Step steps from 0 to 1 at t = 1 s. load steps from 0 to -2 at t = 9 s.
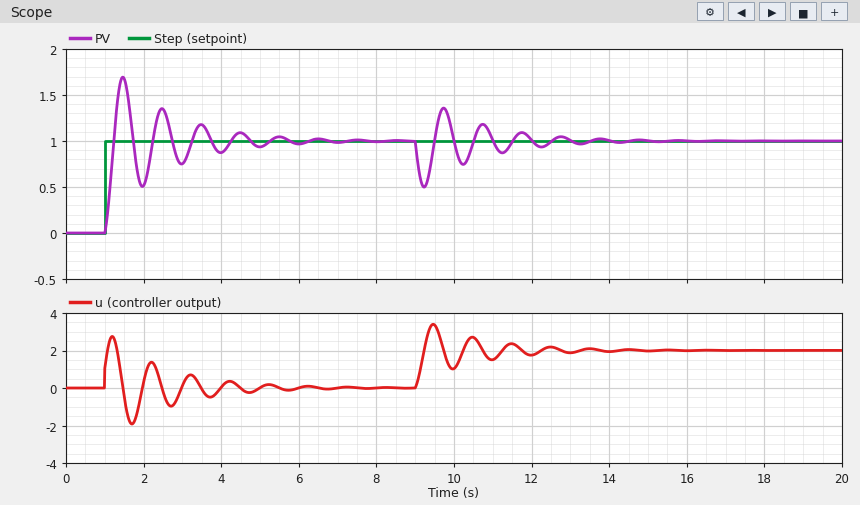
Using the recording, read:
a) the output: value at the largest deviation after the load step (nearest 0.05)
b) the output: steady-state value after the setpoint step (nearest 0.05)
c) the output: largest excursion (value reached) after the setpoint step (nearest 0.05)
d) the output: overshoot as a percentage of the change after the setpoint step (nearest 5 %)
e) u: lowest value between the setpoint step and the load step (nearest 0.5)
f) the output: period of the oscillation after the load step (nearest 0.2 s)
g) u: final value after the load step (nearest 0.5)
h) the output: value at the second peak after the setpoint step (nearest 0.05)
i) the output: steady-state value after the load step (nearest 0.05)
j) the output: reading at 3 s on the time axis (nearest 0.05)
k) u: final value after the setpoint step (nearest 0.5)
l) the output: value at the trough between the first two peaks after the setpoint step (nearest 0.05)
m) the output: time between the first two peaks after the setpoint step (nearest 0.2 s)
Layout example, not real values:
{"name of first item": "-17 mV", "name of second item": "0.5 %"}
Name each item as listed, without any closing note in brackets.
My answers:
{"the output: value at the largest deviation after the load step": "0.50", "the output: steady-state value after the setpoint step": "1.00", "the output: largest excursion (value reached) after the setpoint step": "1.70", "the output: overshoot as a percentage of the change after the setpoint step": "70 %", "u: lowest value between the setpoint step and the load step": "-2.0", "the output: period of the oscillation after the load step": "1.0 s", "u: final value after the load step": "2.0", "the output: value at the second peak after the setpoint step": "1.35", "the output: steady-state value after the load step": "1.00", "the output: reading at 3 s on the time axis": "0.75", "u: final value after the setpoint step": "0.0", "the output: value at the trough between the first two peaks after the setpoint step": "0.50", "the output: time between the first two peaks after the setpoint step": "1.0 s"}
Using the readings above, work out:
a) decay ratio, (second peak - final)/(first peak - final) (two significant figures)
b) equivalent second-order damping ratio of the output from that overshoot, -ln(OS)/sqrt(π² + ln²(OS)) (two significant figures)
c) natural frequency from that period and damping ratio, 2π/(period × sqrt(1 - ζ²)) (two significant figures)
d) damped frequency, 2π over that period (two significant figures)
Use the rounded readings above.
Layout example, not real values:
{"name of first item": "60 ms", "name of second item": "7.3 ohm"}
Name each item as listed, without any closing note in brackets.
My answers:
{"decay ratio, (second peak - final)/(first peak - final)": "0.50", "equivalent second-order damping ratio of the output from that overshoot, -ln(OS)/sqrt(π² + ln²(OS))": "0.11", "natural frequency from that period and damping ratio, 2π/(period × sqrt(1 - ζ²))": "6.3 rad/s", "damped frequency, 2π over that period": "6.3 rad/s"}
